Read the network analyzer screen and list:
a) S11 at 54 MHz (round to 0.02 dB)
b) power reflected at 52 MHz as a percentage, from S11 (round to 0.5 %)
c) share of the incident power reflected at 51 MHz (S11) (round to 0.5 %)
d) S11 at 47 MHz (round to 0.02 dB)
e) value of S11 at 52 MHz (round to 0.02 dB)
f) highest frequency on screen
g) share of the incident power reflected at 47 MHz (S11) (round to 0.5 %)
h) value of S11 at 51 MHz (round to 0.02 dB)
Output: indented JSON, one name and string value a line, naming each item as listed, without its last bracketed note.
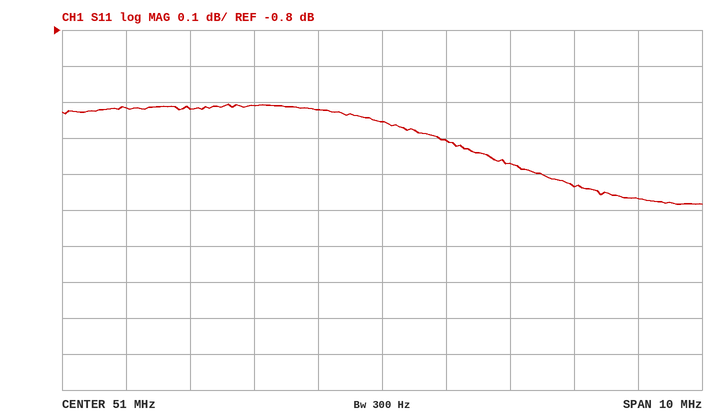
{
  "S11 at 54 MHz": "-1.24 dB",
  "power reflected at 52 MHz as a percentage, from S11": "77.5 %",
  "share of the incident power reflected at 51 MHz (S11)": "78.5 %",
  "S11 at 47 MHz": "-1.02 dB",
  "value of S11 at 52 MHz": "-1.10 dB",
  "highest frequency on screen": "56 MHz",
  "share of the incident power reflected at 47 MHz (S11)": "79.0 %",
  "value of S11 at 51 MHz": "-1.06 dB"
}
